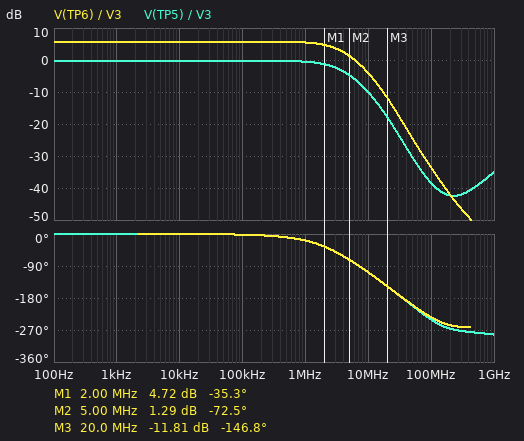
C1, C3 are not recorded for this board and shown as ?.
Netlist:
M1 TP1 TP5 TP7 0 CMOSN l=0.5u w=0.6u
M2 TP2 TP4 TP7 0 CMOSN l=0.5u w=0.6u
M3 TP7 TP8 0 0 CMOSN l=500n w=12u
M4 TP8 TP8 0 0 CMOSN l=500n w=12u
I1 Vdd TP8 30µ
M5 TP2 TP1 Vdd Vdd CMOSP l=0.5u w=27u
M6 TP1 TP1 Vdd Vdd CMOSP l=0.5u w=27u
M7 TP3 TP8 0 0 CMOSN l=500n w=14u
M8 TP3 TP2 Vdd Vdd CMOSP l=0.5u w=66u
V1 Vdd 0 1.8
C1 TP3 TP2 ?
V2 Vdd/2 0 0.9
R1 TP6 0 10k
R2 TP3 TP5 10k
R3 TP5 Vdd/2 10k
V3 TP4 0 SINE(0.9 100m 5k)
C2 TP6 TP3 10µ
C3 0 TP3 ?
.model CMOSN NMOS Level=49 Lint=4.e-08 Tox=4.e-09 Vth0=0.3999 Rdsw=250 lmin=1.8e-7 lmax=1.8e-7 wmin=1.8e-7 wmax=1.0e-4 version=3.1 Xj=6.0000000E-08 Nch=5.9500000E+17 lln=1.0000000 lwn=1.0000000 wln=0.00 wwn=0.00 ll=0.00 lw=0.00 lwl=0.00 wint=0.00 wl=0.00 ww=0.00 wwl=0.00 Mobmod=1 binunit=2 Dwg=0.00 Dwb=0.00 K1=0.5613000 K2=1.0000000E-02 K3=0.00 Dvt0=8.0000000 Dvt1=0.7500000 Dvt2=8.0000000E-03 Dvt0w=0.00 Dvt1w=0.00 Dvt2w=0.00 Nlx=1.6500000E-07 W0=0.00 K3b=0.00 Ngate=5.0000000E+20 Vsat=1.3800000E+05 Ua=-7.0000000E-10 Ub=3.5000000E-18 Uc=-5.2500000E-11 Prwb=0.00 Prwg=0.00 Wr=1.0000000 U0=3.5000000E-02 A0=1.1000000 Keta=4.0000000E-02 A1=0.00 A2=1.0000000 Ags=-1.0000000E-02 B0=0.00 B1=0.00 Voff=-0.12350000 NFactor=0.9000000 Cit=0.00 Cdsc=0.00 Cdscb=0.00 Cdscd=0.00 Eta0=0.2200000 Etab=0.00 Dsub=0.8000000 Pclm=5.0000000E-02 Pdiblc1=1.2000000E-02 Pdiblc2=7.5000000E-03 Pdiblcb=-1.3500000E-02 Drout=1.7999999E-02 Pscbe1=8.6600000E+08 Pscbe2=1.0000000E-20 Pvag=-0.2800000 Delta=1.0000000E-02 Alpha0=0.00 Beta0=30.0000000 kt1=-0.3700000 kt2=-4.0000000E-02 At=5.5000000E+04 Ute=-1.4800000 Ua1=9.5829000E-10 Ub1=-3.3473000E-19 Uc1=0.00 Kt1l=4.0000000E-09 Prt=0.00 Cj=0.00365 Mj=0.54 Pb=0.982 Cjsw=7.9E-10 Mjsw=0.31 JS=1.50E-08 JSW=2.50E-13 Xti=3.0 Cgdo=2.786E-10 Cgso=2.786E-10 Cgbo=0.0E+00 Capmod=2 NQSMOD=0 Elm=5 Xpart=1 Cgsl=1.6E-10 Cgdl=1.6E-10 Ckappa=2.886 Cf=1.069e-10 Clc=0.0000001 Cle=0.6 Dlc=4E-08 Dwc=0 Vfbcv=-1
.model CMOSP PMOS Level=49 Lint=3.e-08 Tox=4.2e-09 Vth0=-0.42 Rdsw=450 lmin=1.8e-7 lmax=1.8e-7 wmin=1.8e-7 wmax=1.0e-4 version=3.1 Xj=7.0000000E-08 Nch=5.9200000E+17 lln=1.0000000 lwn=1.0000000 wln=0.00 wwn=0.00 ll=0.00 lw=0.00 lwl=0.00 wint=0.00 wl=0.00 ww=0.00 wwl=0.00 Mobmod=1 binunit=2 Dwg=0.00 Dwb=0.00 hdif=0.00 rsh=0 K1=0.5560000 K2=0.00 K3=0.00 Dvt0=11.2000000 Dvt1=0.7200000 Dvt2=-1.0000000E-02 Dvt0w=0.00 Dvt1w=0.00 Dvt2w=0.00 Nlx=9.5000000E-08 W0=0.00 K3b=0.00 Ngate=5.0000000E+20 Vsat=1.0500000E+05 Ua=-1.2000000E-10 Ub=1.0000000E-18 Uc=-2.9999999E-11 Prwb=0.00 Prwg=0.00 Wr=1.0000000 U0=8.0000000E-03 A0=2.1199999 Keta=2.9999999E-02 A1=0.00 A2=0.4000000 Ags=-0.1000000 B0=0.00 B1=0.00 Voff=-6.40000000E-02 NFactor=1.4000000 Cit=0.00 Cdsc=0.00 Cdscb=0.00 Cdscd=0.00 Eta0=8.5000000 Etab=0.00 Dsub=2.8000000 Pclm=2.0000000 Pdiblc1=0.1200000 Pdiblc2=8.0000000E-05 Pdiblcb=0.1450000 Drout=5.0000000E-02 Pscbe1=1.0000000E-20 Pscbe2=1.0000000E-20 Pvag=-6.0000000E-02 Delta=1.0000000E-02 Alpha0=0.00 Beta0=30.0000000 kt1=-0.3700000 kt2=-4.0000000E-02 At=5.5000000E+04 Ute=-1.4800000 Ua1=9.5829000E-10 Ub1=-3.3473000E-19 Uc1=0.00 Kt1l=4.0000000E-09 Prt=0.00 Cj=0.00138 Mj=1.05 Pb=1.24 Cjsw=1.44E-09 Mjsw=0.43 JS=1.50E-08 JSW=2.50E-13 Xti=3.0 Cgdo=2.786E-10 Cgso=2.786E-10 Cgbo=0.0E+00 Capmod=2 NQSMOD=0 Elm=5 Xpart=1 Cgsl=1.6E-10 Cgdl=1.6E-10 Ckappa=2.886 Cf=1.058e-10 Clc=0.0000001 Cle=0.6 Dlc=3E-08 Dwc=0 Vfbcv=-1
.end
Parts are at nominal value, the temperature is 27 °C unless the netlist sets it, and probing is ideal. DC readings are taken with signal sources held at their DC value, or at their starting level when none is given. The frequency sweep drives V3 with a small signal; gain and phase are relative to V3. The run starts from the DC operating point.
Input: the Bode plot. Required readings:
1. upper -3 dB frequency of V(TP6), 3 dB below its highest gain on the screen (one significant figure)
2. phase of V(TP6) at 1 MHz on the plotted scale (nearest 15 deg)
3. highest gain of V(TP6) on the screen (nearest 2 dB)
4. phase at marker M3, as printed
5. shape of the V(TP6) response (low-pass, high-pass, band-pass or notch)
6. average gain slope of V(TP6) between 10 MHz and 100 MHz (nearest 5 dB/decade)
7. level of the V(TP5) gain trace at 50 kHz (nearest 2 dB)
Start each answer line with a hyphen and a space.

- 4 MHz
- -15 deg
- 6 dB
- -146.8 deg
- low-pass
- -30 dB/decade
- 0 dB
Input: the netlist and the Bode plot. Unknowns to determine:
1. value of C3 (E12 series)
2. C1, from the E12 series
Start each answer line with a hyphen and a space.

- 4.7 pF
- 1.5 pF
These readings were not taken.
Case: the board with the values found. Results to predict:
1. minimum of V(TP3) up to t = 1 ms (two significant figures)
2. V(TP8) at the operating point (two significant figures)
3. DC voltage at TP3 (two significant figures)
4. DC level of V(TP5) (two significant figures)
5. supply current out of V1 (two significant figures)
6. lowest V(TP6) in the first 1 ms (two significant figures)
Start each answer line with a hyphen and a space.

- 710 mV
- 550 mV
- 900 mV
- 900 mV
- 93 µA
- -190 mV
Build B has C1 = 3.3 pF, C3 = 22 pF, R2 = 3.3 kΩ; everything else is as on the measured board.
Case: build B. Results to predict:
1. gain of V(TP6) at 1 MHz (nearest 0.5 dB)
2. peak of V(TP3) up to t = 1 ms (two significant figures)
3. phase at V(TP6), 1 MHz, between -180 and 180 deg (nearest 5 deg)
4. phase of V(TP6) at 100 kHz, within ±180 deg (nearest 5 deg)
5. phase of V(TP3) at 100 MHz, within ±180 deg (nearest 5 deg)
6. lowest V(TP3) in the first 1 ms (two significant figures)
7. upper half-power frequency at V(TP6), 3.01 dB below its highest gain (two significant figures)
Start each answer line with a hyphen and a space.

- 2.0 dB
- 1.0 V
- -30 deg
- -5 deg
- 100 deg
- 770 mV
- 3.1 MHz
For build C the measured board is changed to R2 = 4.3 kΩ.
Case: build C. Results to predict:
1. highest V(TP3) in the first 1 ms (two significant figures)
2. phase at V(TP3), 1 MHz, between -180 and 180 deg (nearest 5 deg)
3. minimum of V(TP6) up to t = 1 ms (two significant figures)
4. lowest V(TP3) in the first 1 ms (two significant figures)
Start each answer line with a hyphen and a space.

- 1.0 V
- -15 deg
- -140 mV
- 760 mV
